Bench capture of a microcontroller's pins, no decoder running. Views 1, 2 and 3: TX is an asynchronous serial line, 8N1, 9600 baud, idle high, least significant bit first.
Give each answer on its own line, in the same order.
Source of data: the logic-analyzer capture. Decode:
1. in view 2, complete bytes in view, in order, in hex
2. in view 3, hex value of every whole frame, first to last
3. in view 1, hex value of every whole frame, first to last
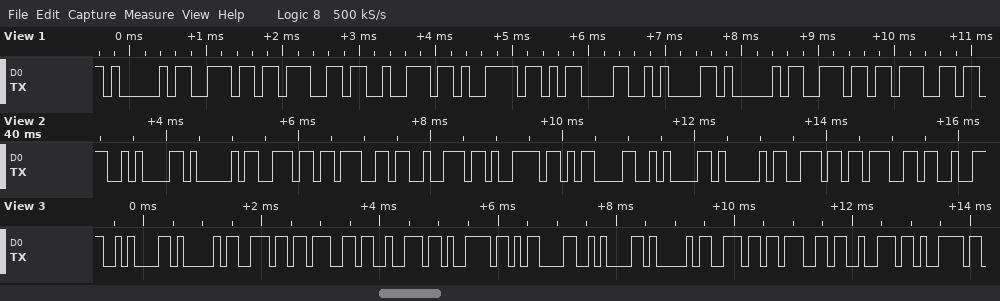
0A 41 6E 67 72 79 0D 0A 41 6E 67
0A 41 6E 67 72 79 0D 0A 41 6E 67 72 79
0x41 0x6E 0x67 0x72 0x79 0x0D 0x0A 0x41 0x6E 0x67
